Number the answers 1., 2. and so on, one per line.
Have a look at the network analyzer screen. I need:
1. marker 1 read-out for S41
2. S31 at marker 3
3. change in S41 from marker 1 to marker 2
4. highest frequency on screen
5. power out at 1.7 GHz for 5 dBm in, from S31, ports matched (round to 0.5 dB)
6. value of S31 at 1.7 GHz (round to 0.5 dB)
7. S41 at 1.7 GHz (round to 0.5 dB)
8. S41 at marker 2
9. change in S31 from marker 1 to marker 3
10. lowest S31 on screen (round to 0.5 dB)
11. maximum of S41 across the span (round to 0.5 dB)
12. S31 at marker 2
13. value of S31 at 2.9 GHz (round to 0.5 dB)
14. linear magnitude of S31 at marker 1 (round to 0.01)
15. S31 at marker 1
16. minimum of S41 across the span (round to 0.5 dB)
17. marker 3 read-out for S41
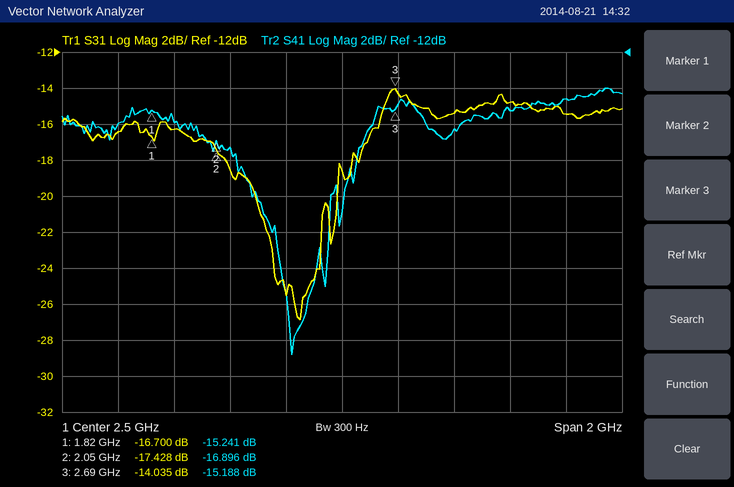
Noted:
1. -15.241 dB
2. -14.035 dB
3. -1.655 dB
4. 3.5 GHz
5. -11.5 dBm
6. -16.5 dB
7. -16.0 dB
8. -16.896 dB
9. 2.665 dB
10. -27.0 dB
11. -14.0 dB
12. -17.428 dB
13. -15.5 dB
14. 0.15
15. -16.700 dB
16. -29.0 dB
17. -15.188 dB
